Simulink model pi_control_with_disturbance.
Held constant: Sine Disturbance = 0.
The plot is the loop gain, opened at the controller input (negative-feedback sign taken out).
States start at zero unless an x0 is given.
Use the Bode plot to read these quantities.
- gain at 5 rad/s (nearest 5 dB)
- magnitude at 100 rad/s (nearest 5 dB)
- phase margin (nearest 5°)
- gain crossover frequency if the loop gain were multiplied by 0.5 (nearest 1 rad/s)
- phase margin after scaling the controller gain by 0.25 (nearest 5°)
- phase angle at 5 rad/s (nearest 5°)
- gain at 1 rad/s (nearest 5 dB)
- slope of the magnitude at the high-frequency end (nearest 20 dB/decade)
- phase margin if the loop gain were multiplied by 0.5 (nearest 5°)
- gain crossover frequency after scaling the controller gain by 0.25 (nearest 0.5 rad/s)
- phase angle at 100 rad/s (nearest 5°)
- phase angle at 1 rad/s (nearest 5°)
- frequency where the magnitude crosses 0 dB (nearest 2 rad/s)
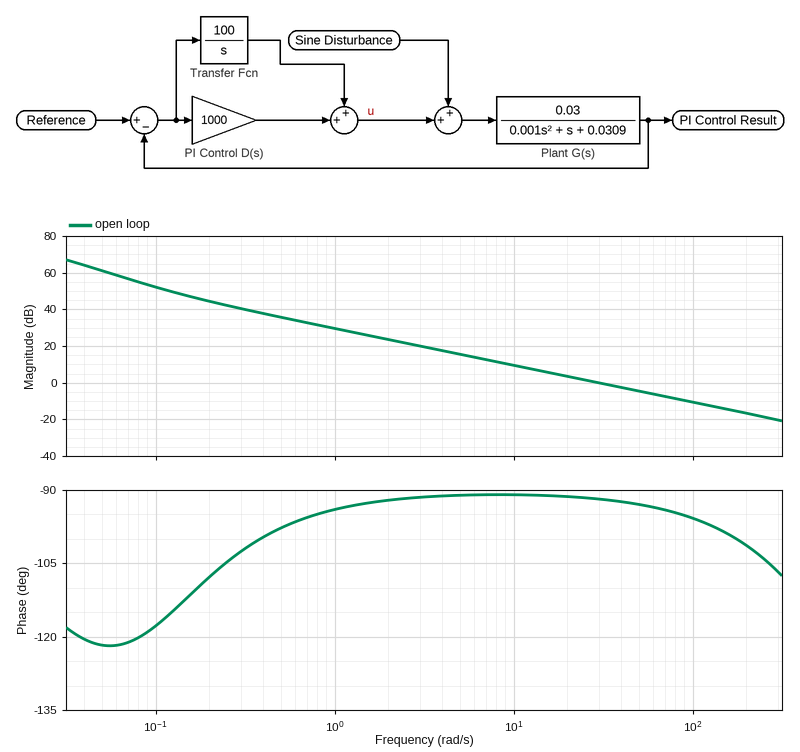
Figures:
15 dB
-10 dB
90°
15 rad/s
90°
-90°
30 dB
-20 dB/decade
90°
7.5 rad/s
-95°
-95°
30 rad/s
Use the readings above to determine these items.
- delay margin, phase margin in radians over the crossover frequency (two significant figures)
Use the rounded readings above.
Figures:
0.052 s
